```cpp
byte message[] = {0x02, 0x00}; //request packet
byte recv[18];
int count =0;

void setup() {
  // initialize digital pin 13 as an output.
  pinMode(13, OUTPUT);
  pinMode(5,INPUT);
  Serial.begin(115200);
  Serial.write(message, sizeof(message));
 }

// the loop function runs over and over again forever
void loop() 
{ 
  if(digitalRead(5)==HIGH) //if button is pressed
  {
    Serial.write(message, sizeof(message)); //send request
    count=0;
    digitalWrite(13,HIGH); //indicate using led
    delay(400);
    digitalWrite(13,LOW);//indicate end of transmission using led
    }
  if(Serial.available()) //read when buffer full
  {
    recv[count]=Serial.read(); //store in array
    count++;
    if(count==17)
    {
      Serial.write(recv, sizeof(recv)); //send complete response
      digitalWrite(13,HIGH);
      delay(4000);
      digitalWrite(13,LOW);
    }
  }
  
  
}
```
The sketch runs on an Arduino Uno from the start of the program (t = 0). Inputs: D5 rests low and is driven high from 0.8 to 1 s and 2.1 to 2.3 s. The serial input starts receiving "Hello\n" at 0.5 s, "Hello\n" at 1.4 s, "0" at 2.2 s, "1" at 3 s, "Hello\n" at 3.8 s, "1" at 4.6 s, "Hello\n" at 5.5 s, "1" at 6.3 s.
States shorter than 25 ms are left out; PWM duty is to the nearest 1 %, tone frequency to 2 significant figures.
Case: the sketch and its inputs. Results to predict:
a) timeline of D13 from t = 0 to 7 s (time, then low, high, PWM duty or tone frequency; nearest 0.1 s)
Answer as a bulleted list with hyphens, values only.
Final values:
- 0 s low; 0.8 s high; 1.2 s low; 2.1 s high; 2.5 s low
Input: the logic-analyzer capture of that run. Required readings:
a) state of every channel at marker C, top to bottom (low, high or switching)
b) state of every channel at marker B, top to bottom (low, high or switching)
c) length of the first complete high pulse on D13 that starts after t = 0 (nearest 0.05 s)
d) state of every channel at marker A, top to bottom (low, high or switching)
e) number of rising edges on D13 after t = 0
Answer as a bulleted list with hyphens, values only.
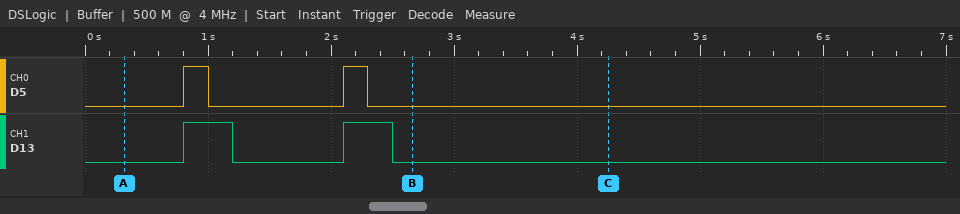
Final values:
- D5 low, D13 low
- D5 low, D13 low
- 0.40 s
- D5 low, D13 low
- 2
